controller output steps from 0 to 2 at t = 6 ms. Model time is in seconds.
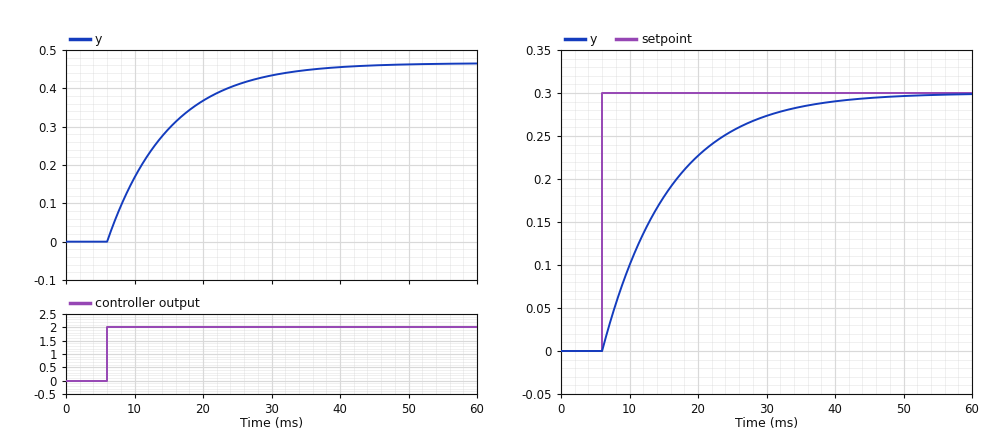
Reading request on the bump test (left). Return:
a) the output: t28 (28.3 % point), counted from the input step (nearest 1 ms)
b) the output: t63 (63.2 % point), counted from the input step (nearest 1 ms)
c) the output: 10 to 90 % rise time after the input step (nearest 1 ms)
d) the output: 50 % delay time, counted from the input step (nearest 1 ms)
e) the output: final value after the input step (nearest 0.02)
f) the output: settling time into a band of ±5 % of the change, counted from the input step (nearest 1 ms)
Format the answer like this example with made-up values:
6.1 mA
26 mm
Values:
3 ms
9 ms
20 ms
6 ms
0.46
27 ms
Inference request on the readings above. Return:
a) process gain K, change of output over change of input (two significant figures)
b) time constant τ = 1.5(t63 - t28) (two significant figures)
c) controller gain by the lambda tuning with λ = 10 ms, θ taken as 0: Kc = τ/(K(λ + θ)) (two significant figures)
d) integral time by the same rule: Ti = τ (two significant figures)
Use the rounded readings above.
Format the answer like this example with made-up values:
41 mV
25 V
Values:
0.23
9.0 ms
3.9
9.0 ms
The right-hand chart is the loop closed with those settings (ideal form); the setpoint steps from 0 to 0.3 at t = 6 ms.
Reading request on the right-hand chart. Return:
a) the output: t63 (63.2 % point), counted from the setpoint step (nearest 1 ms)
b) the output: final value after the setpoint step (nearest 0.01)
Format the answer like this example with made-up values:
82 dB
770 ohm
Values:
10 ms
0.30
